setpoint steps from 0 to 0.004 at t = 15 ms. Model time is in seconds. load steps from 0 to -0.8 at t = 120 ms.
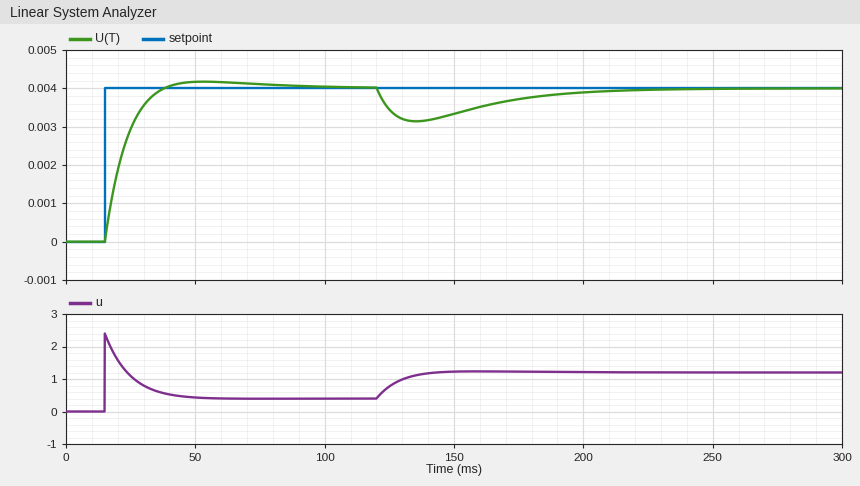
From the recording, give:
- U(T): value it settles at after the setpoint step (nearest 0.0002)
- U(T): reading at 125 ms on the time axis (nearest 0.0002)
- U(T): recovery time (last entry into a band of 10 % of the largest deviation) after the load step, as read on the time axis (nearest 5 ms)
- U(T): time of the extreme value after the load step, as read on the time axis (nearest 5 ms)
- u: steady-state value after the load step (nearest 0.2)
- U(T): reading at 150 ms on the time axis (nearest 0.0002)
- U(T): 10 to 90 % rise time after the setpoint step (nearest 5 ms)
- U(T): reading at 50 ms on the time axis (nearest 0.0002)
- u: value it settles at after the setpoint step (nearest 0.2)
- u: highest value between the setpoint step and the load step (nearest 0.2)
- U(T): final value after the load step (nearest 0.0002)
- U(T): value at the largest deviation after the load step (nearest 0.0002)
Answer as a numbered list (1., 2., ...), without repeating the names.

1. 0.0040
2. 0.0034
3. 205 ms
4. 135 ms
5. 1.2
6. 0.0034
7. 15 ms
8. 0.0042
9. 0.4
10. 2.4
11. 0.0040
12. 0.0032
